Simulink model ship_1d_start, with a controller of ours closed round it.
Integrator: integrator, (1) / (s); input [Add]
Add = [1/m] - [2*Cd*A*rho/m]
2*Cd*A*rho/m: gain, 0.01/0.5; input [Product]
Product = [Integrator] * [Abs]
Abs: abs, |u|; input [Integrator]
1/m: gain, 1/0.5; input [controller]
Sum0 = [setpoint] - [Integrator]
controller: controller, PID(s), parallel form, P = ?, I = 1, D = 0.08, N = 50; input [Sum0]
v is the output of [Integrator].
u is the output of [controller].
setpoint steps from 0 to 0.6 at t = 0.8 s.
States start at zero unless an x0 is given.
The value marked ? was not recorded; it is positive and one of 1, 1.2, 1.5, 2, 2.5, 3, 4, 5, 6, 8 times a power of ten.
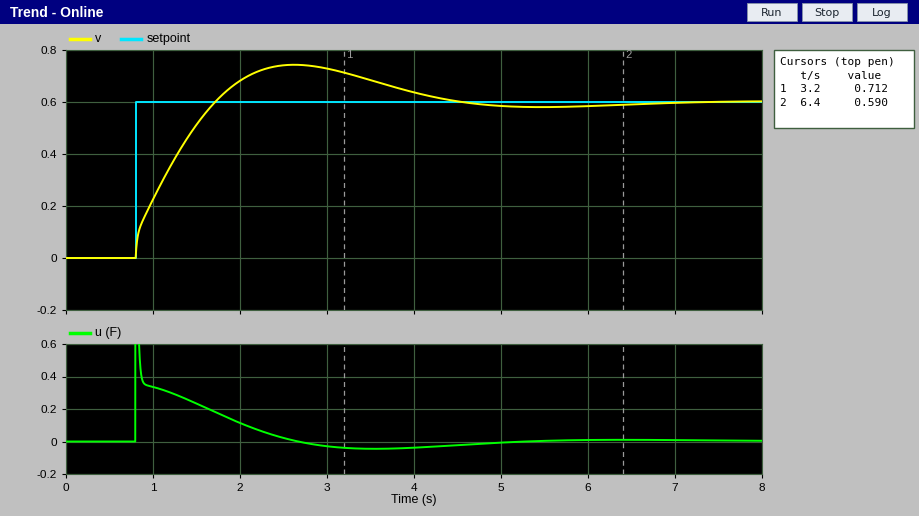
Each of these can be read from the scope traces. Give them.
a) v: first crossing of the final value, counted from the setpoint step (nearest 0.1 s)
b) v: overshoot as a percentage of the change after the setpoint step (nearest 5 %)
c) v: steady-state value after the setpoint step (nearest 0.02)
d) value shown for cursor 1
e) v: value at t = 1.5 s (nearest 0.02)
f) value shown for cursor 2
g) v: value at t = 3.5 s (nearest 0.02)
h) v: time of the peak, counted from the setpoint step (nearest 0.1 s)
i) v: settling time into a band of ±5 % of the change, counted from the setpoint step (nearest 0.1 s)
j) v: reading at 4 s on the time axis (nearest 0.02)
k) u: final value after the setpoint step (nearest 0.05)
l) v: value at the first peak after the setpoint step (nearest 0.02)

0.9 s
25 %
0.60
0.712
0.52
0.590
0.68
1.8 s
3.3 s
0.64
0.00
0.74
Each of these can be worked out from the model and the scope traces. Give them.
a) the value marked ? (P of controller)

0.8
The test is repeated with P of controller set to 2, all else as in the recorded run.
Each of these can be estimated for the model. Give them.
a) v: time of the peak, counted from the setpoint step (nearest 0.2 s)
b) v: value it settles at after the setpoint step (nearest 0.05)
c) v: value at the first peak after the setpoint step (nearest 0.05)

1.4 s
0.60
0.65
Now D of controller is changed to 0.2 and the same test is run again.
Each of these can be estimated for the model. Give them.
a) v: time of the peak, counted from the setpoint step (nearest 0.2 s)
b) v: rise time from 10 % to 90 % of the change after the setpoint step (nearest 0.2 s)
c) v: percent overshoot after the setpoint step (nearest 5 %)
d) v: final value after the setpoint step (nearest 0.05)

2.0 s
0.8 s
20 %
0.60
